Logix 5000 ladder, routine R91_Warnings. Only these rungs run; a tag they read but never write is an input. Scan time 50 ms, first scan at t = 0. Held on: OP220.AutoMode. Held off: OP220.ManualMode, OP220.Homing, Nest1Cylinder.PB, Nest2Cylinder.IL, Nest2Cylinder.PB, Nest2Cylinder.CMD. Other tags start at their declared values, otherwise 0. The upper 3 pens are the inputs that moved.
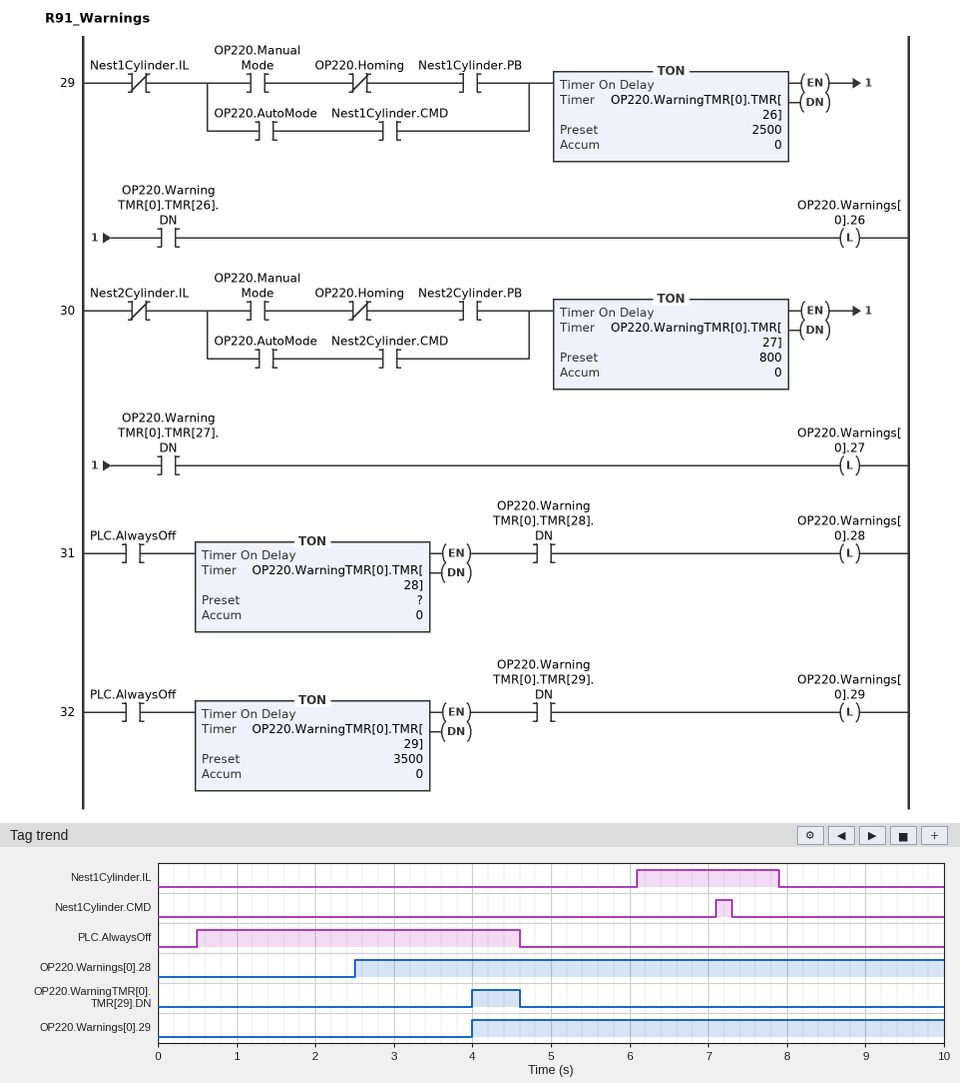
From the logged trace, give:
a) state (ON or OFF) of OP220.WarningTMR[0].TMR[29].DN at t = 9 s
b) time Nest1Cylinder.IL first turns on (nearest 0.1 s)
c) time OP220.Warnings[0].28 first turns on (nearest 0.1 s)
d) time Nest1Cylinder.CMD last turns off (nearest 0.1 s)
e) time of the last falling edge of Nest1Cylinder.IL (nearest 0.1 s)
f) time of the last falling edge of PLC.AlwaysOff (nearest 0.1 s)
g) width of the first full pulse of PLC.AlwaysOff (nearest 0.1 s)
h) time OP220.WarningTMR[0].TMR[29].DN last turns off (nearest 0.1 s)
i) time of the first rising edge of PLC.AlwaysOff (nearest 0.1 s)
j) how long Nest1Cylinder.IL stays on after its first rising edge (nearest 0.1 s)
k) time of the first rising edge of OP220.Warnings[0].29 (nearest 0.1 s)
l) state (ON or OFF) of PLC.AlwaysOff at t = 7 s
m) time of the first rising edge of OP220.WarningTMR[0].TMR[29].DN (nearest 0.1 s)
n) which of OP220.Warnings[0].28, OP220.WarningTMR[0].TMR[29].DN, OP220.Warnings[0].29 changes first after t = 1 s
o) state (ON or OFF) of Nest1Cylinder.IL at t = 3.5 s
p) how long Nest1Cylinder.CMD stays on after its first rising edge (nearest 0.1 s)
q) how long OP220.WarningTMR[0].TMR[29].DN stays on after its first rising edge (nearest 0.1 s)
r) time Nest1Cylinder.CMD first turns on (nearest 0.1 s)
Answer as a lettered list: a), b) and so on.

a) OFF
b) 6.1 s
c) 2.5 s
d) 7.3 s
e) 7.9 s
f) 4.6 s
g) 4.1 s
h) 4.6 s
i) 0.5 s
j) 1.8 s
k) 4.0 s
l) OFF
m) 4.0 s
n) OP220.Warnings[0].28
o) OFF
p) 0.2 s
q) 0.6 s
r) 7.1 s
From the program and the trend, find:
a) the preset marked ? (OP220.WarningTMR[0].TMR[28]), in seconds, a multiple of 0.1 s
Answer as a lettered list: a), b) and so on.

a) 2.0 s
